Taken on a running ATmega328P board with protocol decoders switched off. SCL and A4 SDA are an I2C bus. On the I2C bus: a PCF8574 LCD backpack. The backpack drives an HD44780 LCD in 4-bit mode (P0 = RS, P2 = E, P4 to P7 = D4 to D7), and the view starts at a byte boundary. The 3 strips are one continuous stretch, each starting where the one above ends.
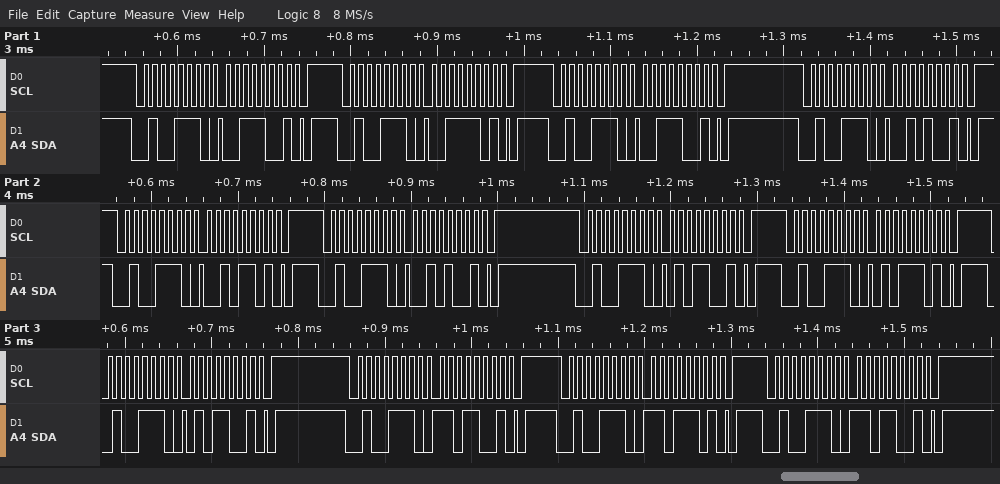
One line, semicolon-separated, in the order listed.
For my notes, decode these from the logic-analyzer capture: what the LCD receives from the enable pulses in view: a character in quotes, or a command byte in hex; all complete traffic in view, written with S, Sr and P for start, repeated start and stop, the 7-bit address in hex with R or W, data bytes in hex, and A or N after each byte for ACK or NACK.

'2' ']'; S 27W A 39 A P S 27W A 3D A P S 27W A 39 A P S 27W A 29 A P S 27W A 2D A P S 27W A 29 A P S 27W A 59 A P S 27W A 5D A P S 27W A 59 A P S 27W A D9 A P S 27W A DD A P S 27W A D9 A P
